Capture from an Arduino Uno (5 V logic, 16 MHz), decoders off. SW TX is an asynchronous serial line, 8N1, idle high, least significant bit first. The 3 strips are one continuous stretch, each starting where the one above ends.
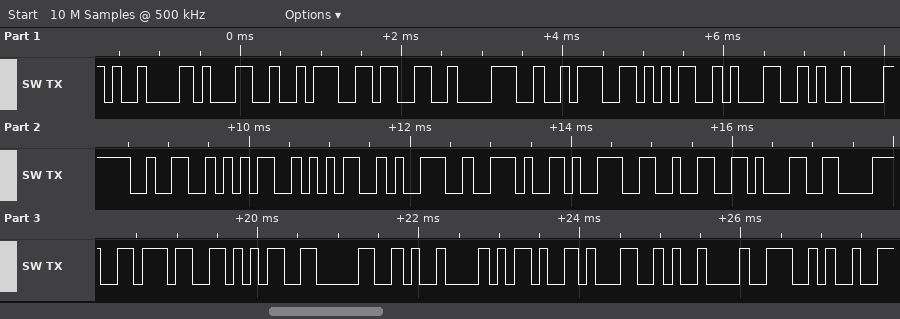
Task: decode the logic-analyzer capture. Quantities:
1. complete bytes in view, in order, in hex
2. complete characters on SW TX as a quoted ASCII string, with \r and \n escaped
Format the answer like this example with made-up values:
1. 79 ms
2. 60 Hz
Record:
1. 09 31 3A 33 38 3A 35 31 09 32 35 35 39 2E 39 32 31 38 37 35 30 09 2D 31 09 4E
2. "\t1:38:51\t2559.9218750\t-1\tN"
